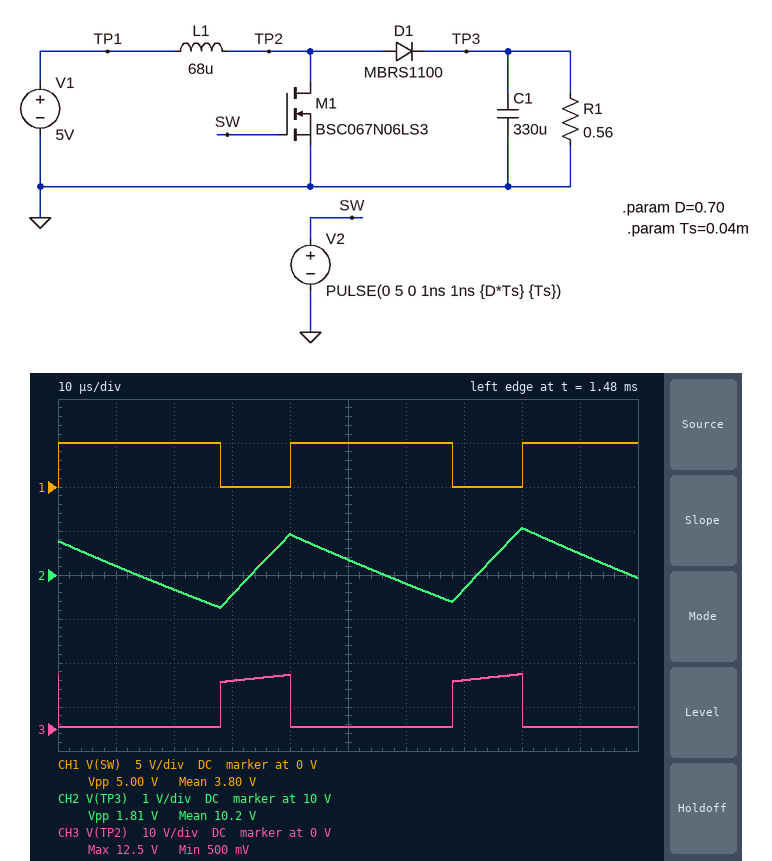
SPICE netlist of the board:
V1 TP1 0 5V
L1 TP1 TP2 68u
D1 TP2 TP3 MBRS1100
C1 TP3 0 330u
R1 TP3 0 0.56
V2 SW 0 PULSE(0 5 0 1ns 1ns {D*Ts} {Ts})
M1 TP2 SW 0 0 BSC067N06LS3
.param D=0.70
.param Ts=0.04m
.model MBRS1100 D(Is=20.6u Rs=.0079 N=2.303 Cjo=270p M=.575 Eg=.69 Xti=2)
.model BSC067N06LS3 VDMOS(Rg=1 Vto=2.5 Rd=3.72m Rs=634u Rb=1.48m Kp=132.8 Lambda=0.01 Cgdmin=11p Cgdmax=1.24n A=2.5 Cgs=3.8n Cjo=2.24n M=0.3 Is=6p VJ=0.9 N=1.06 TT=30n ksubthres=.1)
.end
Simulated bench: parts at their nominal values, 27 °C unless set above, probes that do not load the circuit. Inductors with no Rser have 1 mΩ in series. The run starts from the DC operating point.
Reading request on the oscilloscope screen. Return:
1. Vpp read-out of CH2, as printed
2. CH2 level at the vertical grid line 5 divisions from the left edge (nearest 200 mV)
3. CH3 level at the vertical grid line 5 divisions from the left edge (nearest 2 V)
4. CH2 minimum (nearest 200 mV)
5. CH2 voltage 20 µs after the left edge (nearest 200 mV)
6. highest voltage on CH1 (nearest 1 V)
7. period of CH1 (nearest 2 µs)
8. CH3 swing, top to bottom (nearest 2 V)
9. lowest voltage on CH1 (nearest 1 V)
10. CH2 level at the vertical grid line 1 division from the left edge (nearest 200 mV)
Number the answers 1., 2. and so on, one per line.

1. 1.81 V
2. 10.4 V
3. 0 V
4. 9.2 V
5. 9.6 V
6. 5 V
7. 40 µs
8. 12 V
9. 0 V
10. 10.2 V
